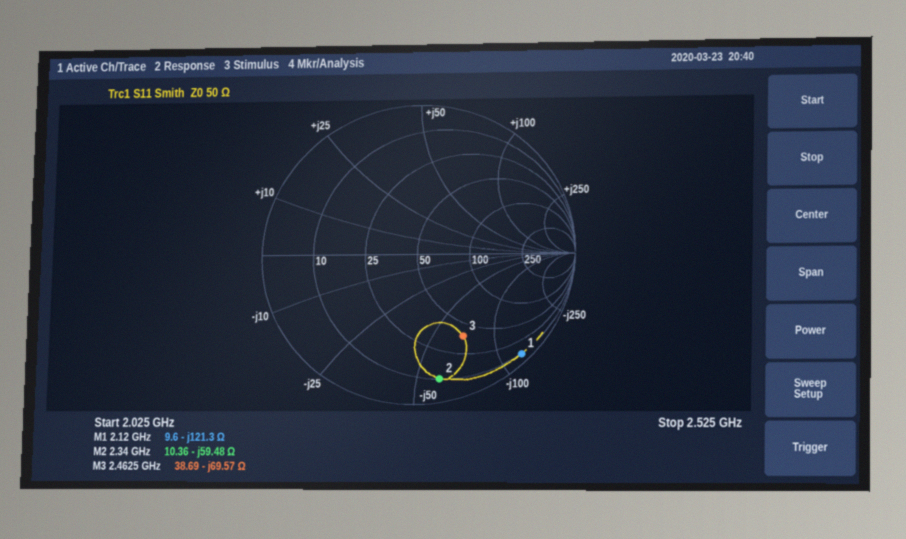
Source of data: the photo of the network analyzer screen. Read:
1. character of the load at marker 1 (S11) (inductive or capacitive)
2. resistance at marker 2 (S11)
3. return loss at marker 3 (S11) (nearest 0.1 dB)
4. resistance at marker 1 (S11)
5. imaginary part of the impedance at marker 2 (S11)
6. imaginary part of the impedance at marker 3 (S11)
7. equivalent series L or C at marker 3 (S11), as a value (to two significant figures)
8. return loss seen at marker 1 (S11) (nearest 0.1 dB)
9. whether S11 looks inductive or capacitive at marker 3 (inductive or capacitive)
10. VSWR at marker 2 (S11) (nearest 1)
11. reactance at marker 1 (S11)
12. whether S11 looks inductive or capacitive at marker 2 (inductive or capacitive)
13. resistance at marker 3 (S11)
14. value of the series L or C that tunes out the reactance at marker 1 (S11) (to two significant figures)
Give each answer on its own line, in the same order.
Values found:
capacitive
10.36 Ω
4.1 dB
9.6 Ω
-59.48 Ω
-69.57 Ω
930 fF
0.5 dB
capacitive
12
-121.3 Ω
capacitive
38.69 Ω
9.1 nH
